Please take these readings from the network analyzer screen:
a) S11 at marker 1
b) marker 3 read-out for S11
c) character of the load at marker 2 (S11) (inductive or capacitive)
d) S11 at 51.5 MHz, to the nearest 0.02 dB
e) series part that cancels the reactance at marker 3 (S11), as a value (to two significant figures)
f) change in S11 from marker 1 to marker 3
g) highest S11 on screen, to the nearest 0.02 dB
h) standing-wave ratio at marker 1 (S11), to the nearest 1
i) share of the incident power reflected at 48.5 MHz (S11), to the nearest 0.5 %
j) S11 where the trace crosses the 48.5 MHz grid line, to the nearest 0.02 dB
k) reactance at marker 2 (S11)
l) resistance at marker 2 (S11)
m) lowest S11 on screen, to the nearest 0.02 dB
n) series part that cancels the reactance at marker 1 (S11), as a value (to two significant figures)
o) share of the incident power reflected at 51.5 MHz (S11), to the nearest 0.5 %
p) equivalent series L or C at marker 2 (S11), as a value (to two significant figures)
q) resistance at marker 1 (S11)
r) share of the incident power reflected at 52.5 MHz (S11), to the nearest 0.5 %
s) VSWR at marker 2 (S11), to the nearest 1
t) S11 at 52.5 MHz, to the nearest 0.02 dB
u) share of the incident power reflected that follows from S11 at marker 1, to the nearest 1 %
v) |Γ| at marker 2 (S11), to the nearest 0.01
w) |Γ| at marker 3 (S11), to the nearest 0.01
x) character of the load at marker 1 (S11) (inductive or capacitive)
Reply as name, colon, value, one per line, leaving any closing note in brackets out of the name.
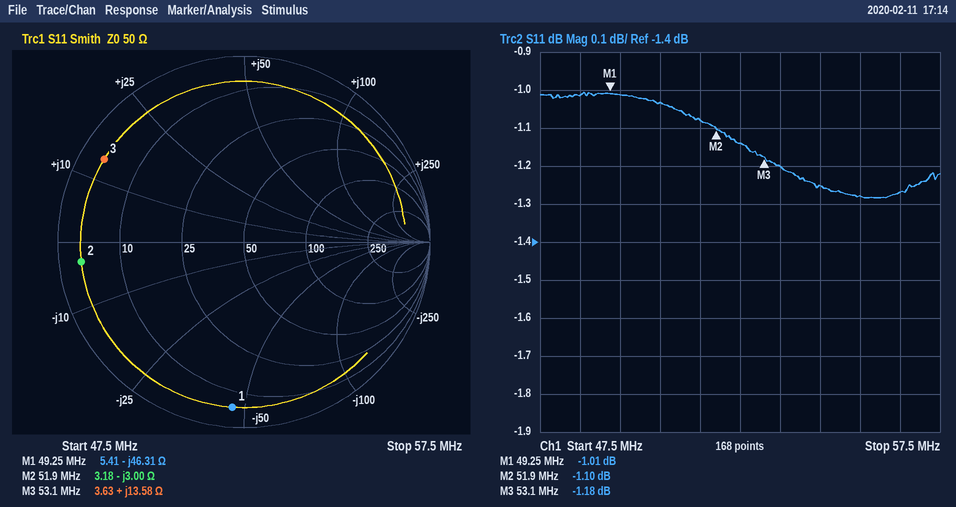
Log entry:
S11 at marker 1: -1.01 dB
marker 3 read-out for S11: -1.18 dB
character of the load at marker 2 (S11): capacitive
S11 at 51.5 MHz, to the nearest 0.02 dB: -1.08 dB
series part that cancels the reactance at marker 3 (S11), as a value: 220 pF
change in S11 from marker 1 to marker 3: -0.17 dB
highest S11 on screen, to the nearest 0.02 dB: -1.00 dB
standing-wave ratio at marker 1 (S11), to the nearest 1: 17
share of the incident power reflected at 48.5 MHz (S11), to the nearest 0.5 %: 79.0 %
S11 where the trace crosses the 48.5 MHz grid line, to the nearest 0.02 dB: -1.02 dB
reactance at marker 2: -3.00 Ω
resistance at marker 2: 3.18 Ω
lowest S11 on screen, to the nearest 0.02 dB: -1.28 dB
series part that cancels the reactance at marker 1 (S11), as a value: 150 nH
share of the incident power reflected at 51.5 MHz (S11), to the nearest 0.5 %: 78.0 %
equivalent series L or C at marker 2 (S11), as a value: 1.0 nF
resistance at marker 1: 5.41 Ω
share of the incident power reflected at 52.5 MHz (S11), to the nearest 0.5 %: 77.0 %
VSWR at marker 2 (S11), to the nearest 1: 16
S11 at 52.5 MHz, to the nearest 0.02 dB: -1.14 dB
share of the incident power reflected that follows from S11 at marker 1, to the nearest 1 %: 79 %
|Γ| at marker 2 (S11), to the nearest 0.01: 0.88
|Γ| at marker 3 (S11), to the nearest 0.01: 0.87
character of the load at marker 1 (S11): capacitive
